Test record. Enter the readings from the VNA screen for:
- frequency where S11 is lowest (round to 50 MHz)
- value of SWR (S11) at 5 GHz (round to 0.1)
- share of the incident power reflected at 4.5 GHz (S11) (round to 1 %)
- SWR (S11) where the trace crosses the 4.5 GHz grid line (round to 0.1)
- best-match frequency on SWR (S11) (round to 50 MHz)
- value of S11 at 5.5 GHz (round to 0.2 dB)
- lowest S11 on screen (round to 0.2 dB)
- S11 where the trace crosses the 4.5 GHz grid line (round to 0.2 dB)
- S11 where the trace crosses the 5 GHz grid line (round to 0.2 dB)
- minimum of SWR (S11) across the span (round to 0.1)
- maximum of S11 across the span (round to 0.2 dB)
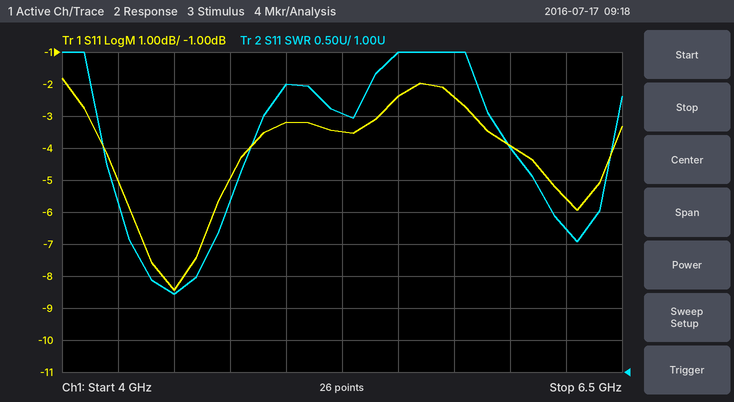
4.50 GHz
5.5
14 %
2.2
4.50 GHz
-2.4 dB
-8.4 dB
-8.4 dB
-3.2 dB
2.2
-1.8 dB
